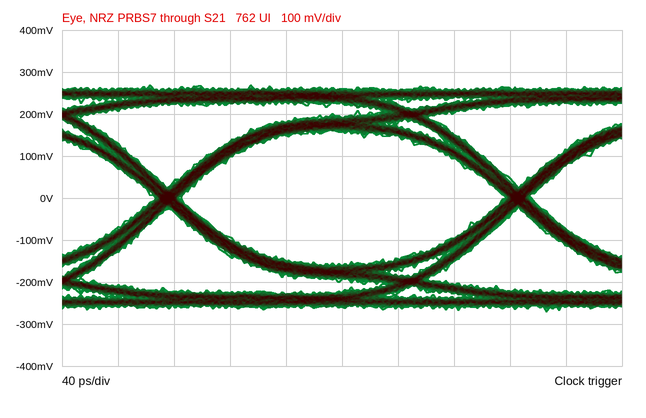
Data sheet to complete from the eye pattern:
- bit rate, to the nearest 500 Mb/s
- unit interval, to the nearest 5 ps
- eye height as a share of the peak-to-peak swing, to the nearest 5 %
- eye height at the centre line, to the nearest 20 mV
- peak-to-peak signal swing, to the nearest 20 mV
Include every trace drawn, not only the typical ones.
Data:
4.0 Gb/s
250 ps
60 %
320 mV
540 mV
